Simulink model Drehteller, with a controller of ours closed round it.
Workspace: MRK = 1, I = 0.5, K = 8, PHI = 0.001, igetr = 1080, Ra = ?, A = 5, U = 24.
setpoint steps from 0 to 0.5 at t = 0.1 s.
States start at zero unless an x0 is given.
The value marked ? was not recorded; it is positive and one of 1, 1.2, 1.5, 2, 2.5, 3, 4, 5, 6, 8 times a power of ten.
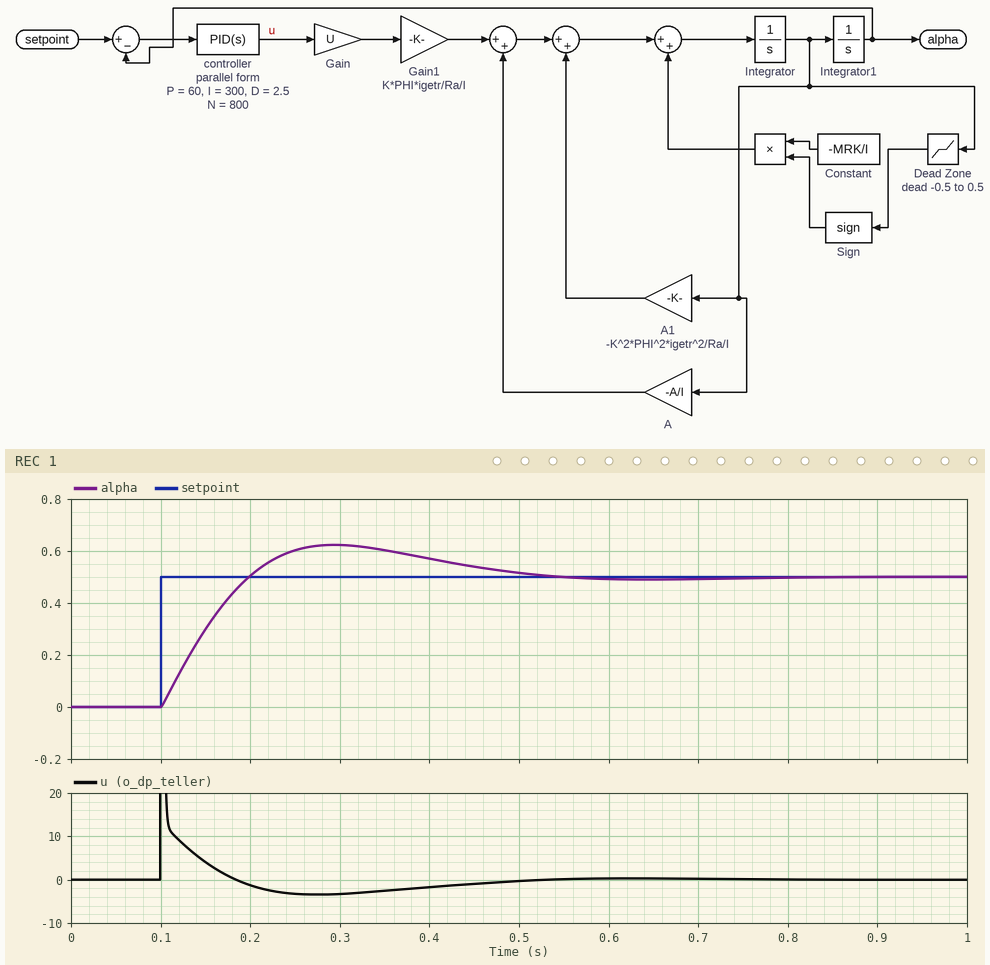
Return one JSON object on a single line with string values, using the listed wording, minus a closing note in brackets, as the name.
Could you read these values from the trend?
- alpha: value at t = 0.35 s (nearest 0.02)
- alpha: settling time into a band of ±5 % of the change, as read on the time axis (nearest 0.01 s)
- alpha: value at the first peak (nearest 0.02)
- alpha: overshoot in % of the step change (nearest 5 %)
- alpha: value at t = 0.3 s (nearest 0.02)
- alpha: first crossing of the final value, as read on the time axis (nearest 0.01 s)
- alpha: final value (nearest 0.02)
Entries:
{"alpha: value at t = 0.35 s": "0.60", "alpha: settling time into a band of ±5 % of the change, as read on the time axis": "0.48 s", "alpha: value at the first peak": "0.62", "alpha: overshoot in % of the step change": "25 %", "alpha: value at t = 0.3 s": "0.62", "alpha: first crossing of the final value, as read on the time axis": "0.20 s", "alpha: final value": "0.50"}
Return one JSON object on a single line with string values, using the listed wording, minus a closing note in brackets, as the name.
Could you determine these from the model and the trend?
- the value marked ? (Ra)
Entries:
{"the value marked ?": "80"}
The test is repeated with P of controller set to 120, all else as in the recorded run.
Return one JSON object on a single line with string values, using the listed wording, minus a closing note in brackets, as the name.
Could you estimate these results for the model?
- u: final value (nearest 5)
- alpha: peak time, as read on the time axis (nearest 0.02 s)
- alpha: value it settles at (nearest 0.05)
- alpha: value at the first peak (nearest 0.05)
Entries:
{"u: final value": "0", "alpha: peak time, as read on the time axis": "0.22 s", "alpha: value it settles at": "0.50", "alpha: value at the first peak": "0.65"}
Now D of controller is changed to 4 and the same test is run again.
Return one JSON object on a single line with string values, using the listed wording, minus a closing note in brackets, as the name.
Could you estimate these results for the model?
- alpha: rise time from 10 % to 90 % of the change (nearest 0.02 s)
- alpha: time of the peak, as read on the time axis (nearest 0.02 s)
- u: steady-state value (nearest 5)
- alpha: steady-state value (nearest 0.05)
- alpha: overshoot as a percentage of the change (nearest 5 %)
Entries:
{"alpha: rise time from 10 % to 90 % of the change": "0.08 s", "alpha: time of the peak, as read on the time axis": "0.32 s", "u: steady-state value": "0", "alpha: steady-state value": "0.50", "alpha: overshoot as a percentage of the change": "15 %"}
